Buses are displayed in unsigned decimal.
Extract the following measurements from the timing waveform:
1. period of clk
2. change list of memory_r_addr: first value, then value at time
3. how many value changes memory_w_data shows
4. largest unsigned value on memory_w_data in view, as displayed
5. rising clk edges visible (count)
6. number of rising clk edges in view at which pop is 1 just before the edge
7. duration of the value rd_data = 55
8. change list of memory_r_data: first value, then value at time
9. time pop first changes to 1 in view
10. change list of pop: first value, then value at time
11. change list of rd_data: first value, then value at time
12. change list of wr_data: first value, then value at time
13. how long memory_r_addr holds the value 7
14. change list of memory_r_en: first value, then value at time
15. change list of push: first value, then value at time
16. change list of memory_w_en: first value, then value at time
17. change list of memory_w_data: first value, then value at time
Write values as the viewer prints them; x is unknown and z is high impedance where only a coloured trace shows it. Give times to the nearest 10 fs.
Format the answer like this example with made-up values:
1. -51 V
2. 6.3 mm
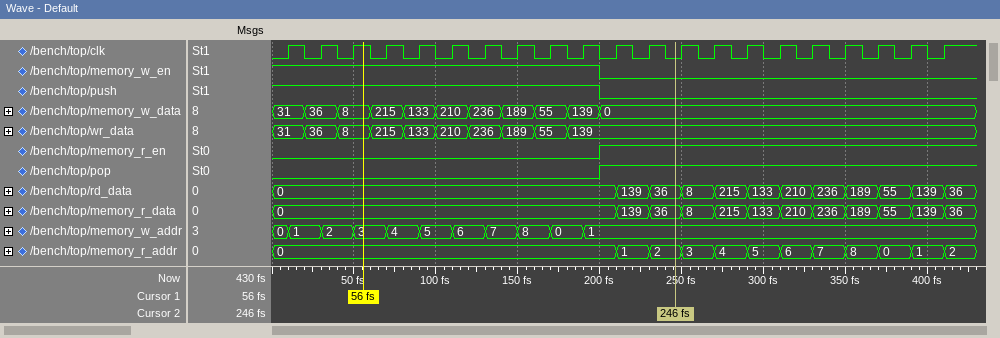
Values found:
1. 20 fs
2. 0, 1 at 210 fs, 2 at 230 fs, 3 at 250 fs, 4 at 270 fs, 5 at 290 fs, 6 at 310 fs, 7 at 330 fs, 8 at 350 fs, 0 at 370 fs, 1 at 390 fs, 2 at 410 fs
3. 10
4. 236
5. 21
6. 11
7. 20 fs
8. 0, 139 at 210 fs, 36 at 230 fs, 8 at 250 fs, 215 at 270 fs, 133 at 290 fs, 210 at 310 fs, 236 at 330 fs, 189 at 350 fs, 55 at 370 fs, 139 at 390 fs, 36 at 410 fs
9. 200 fs
10. 0, 1 at 200 fs
11. 0, 139 at 210 fs, 36 at 230 fs, 8 at 250 fs, 215 at 270 fs, 133 at 290 fs, 210 at 310 fs, 236 at 330 fs, 189 at 350 fs, 55 at 370 fs, 139 at 390 fs, 36 at 410 fs
12. 31, 36 at 20 fs, 8 at 40 fs, 215 at 60 fs, 133 at 80 fs, 210 at 100 fs, 236 at 120 fs, 189 at 140 fs, 55 at 160 fs, 139 at 180 fs
13. 20 fs
14. 0, 1 at 200 fs
15. 1, 0 at 200 fs
16. 1, 0 at 200 fs
17. 31, 36 at 20 fs, 8 at 40 fs, 215 at 60 fs, 133 at 80 fs, 210 at 100 fs, 236 at 120 fs, 189 at 140 fs, 55 at 160 fs, 139 at 180 fs, 0 at 200 fs
